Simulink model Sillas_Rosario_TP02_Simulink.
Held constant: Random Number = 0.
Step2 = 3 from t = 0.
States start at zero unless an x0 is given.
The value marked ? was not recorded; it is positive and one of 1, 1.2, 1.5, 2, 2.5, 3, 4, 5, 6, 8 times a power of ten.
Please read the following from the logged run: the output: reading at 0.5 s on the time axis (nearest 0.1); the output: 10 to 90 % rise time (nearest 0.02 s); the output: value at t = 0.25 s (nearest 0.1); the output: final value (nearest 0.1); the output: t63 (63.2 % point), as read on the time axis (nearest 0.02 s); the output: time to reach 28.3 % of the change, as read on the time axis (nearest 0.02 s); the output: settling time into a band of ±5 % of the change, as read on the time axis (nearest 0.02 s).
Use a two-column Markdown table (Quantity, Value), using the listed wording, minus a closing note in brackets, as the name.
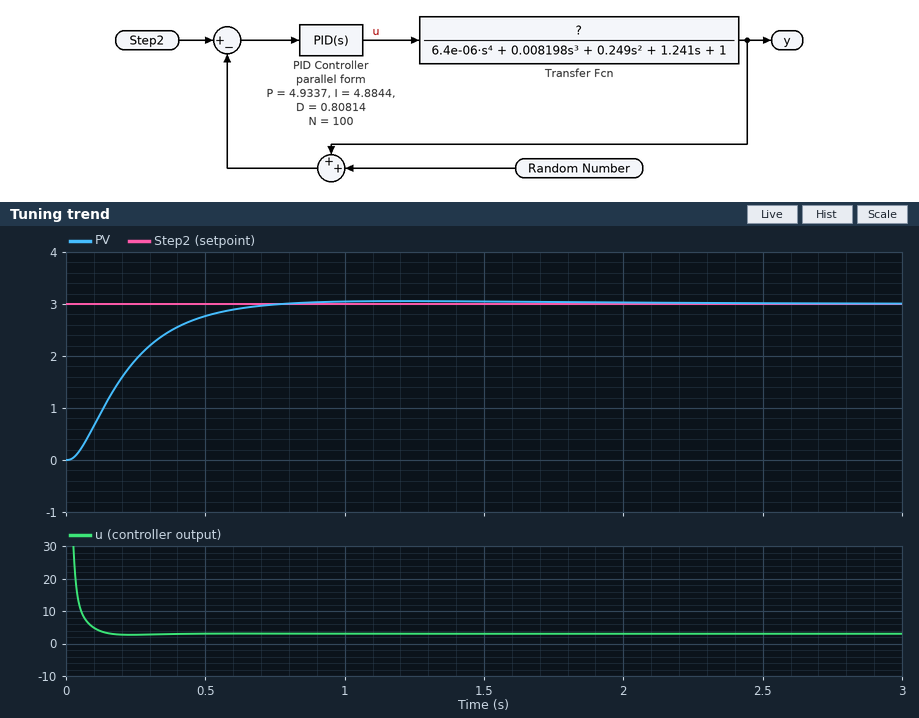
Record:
| Quantity | Value |
|---|---|
| the output: reading at 0.5 s on the time axis | 2.8 |
| the output: 10 to 90 % rise time | 0.40 s |
| the output: value at t = 0.25 s | 1.9 |
| the output: final value | 3.0 |
| the output: t63 (63.2 % point), as read on the time axis | 0.24 s |
| the output: time to reach 28.3 % of the change, as read on the time axis | 0.12 s |
| the output: settling time into a band of ±5 % of the change, as read on the time axis | 0.56 s |
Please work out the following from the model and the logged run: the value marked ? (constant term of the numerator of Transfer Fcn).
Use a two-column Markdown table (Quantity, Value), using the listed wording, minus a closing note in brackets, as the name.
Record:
| Quantity | Value |
|---|---|
| the value marked ? | 1 |
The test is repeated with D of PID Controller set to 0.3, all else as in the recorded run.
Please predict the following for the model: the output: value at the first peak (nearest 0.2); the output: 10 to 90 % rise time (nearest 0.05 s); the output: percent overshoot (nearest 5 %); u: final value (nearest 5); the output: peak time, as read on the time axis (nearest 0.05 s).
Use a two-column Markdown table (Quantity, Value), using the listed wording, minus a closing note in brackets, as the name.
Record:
| Quantity | Value |
|---|---|
| the output: value at the first peak | 3.4 |
| the output: 10 to 90 % rise time | 0.35 s |
| the output: percent overshoot | 10 % |
| u: final value | 5 |
| the output: peak time, as read on the time axis | 0.75 s |
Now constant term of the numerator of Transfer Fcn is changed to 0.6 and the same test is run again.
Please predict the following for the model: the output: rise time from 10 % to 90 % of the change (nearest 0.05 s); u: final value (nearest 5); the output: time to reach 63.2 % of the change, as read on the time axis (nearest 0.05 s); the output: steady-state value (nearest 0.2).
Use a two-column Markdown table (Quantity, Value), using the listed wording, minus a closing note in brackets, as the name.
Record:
| Quantity | Value |
|---|---|
| the output: rise time from 10 % to 90 % of the change | 0.70 s |
| u: final value | 5 |
| the output: time to reach 63.2 % of the change, as read on the time axis | 0.40 s |
| the output: steady-state value | 3.0 |
